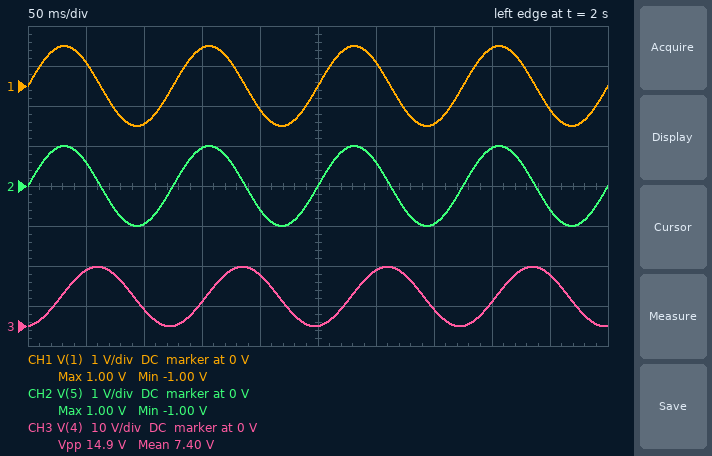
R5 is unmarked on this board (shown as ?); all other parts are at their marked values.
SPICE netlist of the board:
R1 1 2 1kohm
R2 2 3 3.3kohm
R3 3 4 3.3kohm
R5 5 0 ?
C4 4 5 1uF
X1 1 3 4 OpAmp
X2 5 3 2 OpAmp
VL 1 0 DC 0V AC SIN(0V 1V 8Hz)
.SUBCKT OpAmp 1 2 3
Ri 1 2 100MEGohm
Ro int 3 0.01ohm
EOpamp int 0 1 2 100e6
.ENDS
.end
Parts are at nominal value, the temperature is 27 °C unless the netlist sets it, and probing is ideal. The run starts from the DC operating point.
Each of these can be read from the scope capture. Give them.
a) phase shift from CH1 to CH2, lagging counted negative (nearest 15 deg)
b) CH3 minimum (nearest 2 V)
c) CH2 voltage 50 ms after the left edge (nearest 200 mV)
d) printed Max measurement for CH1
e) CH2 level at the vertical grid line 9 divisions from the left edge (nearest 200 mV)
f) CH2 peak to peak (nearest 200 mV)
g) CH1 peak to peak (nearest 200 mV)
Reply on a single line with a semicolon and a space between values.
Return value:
0 deg; 0 V; 600 mV; 1.00 V; -600 mV; 2.0 V; 2.0 V
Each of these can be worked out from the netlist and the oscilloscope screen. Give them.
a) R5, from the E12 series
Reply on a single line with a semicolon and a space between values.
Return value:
2.7 kΩ
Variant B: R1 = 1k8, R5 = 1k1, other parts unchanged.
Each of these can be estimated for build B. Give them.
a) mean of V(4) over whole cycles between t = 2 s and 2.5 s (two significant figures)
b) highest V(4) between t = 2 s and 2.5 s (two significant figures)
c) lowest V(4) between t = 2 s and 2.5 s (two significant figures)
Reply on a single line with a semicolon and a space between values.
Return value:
18 V; 36 V; -28 mV
